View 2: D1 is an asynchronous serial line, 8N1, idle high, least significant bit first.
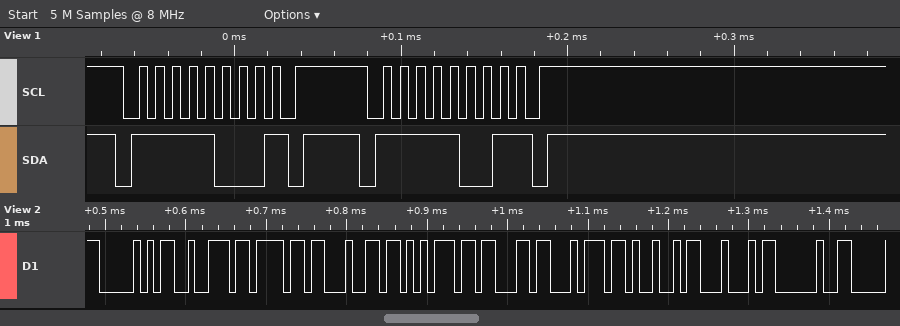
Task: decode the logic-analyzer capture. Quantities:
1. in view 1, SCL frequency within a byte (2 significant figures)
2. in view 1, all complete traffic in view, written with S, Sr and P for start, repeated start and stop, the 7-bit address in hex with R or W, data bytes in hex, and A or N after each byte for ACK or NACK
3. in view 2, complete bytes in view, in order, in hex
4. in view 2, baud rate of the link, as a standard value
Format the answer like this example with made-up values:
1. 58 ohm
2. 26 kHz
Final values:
1. 100 kHz
2. S 7CW N P S 7CR N P
3. 50 72 6F 64 75 63 74 49 44 20
4. 115200 baud
